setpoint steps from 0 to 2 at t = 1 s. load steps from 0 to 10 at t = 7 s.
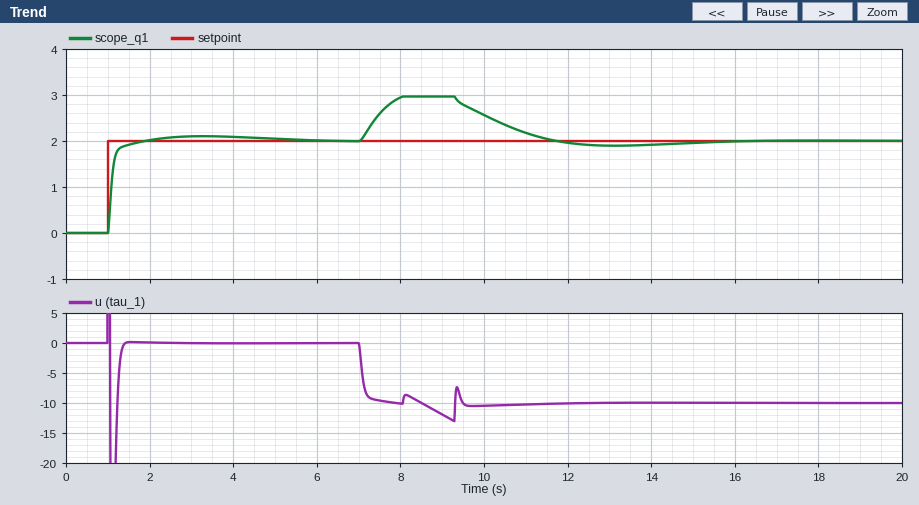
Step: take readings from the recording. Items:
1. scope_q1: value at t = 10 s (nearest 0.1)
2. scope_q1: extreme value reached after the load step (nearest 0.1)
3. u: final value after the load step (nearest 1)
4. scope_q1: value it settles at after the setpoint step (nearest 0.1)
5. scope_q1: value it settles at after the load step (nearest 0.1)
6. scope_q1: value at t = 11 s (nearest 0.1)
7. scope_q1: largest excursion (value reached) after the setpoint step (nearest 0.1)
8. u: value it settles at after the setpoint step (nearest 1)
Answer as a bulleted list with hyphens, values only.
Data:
- 2.6
- 3.0
- -10
- 2.0
- 2.0
- 2.2
- 2.1
- 0
